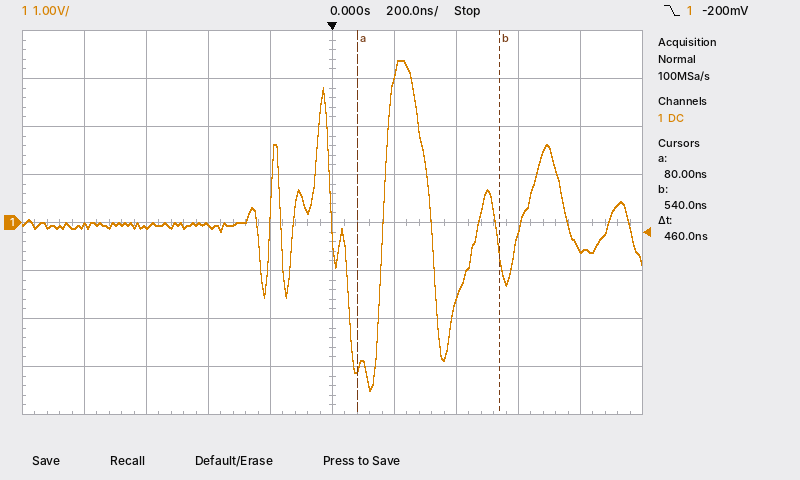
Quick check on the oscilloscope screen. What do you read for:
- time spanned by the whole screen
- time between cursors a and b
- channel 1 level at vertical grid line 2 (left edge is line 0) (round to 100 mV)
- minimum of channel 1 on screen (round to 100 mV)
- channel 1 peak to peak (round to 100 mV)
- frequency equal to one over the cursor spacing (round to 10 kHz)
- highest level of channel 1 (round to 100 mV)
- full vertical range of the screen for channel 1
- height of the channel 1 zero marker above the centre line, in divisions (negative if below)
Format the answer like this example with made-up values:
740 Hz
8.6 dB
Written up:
2 µs
460 ns
-100 mV
-3.5 V
6.9 V
2.17 MHz
3.4 V
8 V
0.0 div
